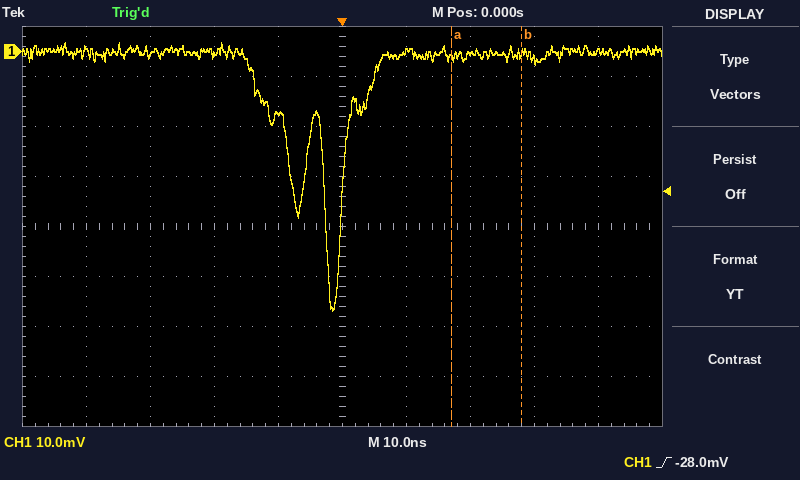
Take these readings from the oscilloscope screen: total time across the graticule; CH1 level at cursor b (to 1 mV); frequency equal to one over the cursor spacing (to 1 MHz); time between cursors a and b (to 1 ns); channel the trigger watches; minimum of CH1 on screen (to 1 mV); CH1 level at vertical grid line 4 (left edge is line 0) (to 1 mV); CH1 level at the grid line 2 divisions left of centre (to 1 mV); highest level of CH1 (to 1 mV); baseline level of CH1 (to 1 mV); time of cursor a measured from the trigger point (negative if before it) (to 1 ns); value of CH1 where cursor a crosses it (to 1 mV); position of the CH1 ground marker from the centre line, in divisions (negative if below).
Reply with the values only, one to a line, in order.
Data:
100 ns
0 mV
91 MHz
11 ns
CH1
-52 mV
-12 mV
0 mV
2 mV
0 mV
+17 ns
-1 mV
+3.5 div
